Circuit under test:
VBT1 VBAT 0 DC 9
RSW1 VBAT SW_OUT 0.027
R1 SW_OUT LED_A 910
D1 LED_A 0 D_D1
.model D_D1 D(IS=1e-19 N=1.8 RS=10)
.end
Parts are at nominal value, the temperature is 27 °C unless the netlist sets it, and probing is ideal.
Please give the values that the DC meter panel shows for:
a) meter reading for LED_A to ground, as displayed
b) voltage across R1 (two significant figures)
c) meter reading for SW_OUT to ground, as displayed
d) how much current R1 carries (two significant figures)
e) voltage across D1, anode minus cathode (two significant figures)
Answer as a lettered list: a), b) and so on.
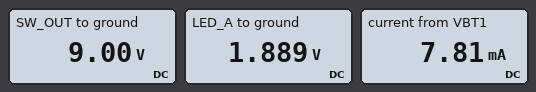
a) 1.889 V
b) 7.1 V
c) 9.00 V
d) 7.8 mA
e) 1.9 V
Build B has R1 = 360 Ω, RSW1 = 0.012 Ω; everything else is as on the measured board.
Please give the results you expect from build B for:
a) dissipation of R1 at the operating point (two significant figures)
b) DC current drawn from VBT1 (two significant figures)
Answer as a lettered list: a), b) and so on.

a) 130 mW
b) 19 mA
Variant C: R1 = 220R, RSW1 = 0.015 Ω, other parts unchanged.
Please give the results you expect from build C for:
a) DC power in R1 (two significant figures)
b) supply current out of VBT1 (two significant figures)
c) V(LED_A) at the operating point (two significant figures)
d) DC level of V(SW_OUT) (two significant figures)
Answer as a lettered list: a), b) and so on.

a) 210 mW
b) 31 mA
c) 2.2 V
d) 9.0 V
